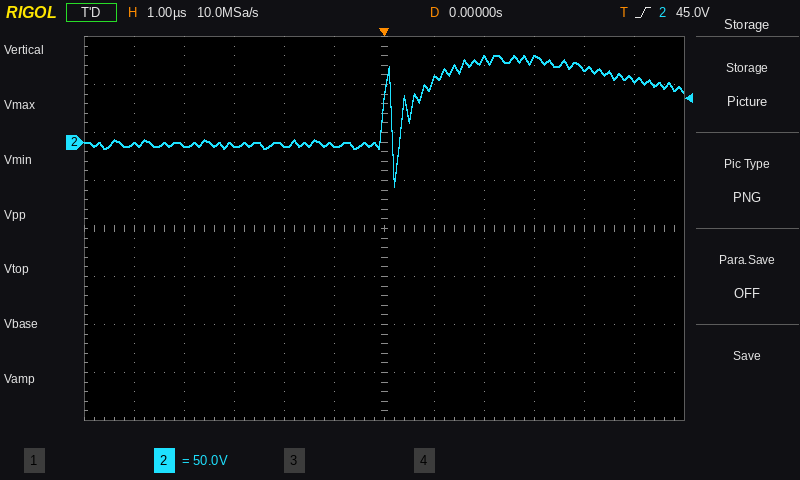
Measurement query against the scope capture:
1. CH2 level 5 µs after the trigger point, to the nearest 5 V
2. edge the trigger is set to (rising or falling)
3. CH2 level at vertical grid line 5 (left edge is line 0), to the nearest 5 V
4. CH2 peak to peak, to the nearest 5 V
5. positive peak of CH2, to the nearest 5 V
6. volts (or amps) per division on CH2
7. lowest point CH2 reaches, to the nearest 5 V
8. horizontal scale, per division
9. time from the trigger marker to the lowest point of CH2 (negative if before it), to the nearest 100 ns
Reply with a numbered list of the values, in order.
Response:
1. 65 V
2. rising
3. -5 V
4. 135 V
5. 90 V
6. 50 V
7. -45 V
8. 1 µs
9. +200 ns
